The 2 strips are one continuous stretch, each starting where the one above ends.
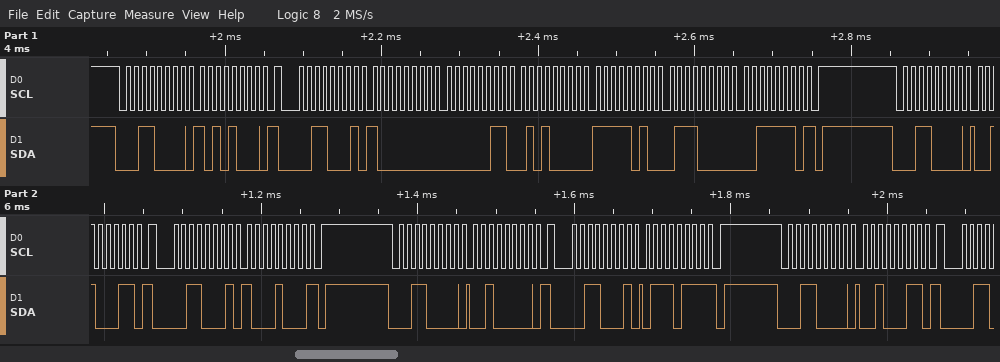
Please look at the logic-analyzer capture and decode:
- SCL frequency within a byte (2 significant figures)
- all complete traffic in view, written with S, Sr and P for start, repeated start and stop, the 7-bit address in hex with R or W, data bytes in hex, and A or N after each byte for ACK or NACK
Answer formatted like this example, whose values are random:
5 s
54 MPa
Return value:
100 kHz
S 18W A A8 A Sr 18R A 80 A 03 A 50 A FA A 70 A 3E N P S 18W A 23 A Sr 18R A 88 N P S 18W A 20 A Sr 18R A 77 N P S 18W A 23 A
